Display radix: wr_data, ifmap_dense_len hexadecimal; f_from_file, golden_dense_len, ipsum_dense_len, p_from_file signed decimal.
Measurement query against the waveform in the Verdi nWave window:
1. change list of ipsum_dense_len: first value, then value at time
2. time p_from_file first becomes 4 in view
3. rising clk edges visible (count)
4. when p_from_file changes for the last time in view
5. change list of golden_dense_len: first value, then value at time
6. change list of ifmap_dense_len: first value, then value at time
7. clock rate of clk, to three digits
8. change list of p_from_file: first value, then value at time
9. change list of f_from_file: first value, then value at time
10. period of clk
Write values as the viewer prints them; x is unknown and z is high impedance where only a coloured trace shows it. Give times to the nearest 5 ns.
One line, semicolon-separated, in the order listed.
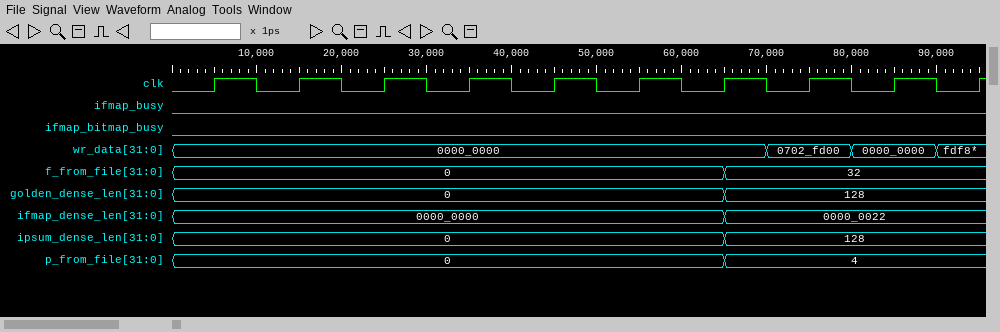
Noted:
0, 128 at 65 ns; 65 ns; 10; 65 ns; 0, 128 at 65 ns; 0000_0000, 0000_0022 at 65 ns; 100 MHz; 0, 4 at 65 ns; 0, 32 at 65 ns; 10 ns
